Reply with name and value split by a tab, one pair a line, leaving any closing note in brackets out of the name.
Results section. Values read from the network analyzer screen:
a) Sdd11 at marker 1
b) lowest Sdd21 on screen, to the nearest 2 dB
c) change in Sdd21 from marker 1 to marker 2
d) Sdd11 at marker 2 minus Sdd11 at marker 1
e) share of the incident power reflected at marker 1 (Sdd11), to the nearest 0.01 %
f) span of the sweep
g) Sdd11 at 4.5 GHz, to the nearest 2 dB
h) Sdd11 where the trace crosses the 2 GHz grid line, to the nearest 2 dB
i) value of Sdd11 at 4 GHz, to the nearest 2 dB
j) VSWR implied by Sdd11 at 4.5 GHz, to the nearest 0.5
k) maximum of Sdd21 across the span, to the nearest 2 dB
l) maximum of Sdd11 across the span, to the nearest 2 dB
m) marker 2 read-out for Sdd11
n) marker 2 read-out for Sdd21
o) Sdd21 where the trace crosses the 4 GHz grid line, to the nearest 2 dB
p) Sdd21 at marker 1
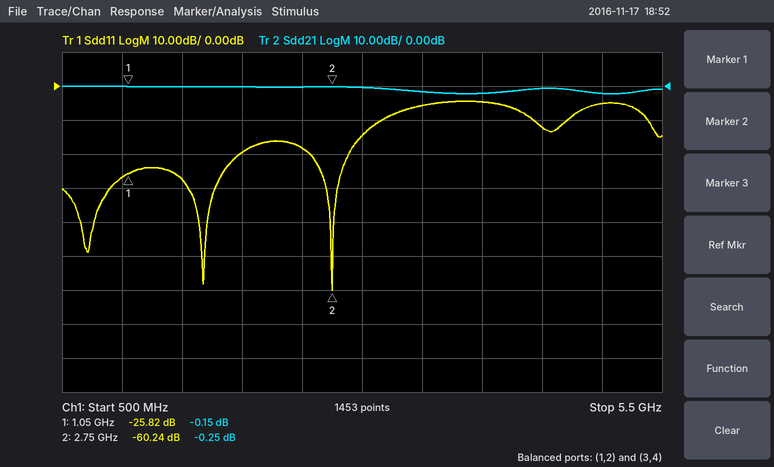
Sdd11 at marker 1	-25.82 dB
lowest Sdd21 on screen, to the nearest 2 dB	-2 dB
change in Sdd21 from marker 1 to marker 2	-0.10 dB
Sdd11 at marker 2 minus Sdd11 at marker 1	-34.42 dB
share of the incident power reflected at marker 1 (Sdd11), to the nearest 0.01 %	0.26 %
span of the sweep	5 GHz
Sdd11 at 4.5 GHz, to the nearest 2 dB	-12 dB
Sdd11 where the trace crosses the 2 GHz grid line, to the nearest 2 dB	-20 dB
value of Sdd11 at 4 GHz, to the nearest 2 dB	-4 dB
VSWR implied by Sdd11 at 4.5 GHz, to the nearest 0.5	1.5
maximum of Sdd21 across the span, to the nearest 2 dB	0 dB
maximum of Sdd11 across the span, to the nearest 2 dB	-4 dB
marker 2 read-out for Sdd11	-60.24 dB
marker 2 read-out for Sdd21	-0.25 dB
Sdd21 where the trace crosses the 4 GHz grid line, to the nearest 2 dB	-2 dB
Sdd21 at marker 1	-0.15 dB
